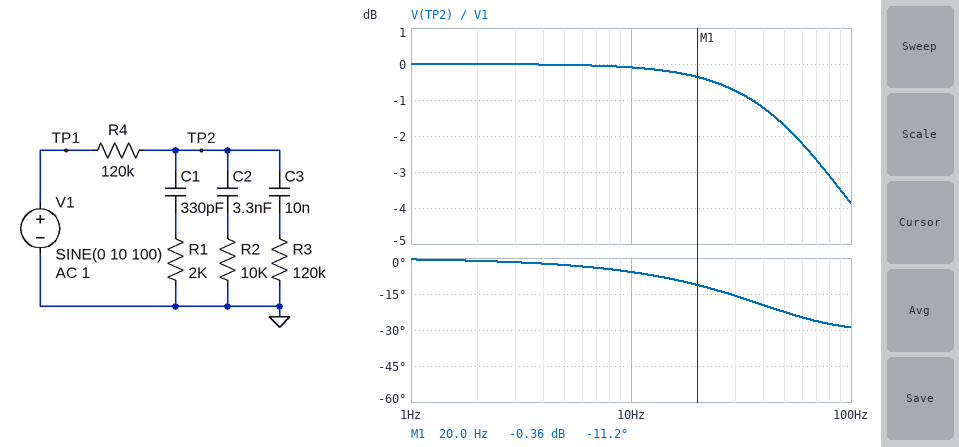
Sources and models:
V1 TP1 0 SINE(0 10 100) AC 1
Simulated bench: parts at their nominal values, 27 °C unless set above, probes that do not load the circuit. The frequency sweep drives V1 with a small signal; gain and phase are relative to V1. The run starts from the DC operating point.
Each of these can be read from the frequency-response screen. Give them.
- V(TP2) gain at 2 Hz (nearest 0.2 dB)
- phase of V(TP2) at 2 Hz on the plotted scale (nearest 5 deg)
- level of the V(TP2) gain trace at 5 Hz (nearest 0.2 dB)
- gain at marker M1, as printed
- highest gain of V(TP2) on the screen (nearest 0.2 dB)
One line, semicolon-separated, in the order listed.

0 dB; 0 deg; 0 dB; -0.36 dB; 0 dB
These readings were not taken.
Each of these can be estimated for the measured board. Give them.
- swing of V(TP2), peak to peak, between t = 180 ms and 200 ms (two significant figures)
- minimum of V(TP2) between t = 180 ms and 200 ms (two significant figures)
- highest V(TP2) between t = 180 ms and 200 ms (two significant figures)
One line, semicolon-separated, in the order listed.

13 V; -6.4 V; 6.4 V
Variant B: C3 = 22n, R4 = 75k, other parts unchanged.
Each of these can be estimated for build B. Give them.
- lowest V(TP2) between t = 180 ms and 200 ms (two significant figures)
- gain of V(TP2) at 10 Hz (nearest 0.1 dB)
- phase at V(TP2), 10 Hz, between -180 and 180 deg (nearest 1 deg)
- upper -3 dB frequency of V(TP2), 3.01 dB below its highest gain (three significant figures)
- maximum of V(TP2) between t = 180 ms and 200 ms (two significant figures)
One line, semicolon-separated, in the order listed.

-6.5 V; -0.2 dB; -7 deg; 67.4 Hz; 6.5 V
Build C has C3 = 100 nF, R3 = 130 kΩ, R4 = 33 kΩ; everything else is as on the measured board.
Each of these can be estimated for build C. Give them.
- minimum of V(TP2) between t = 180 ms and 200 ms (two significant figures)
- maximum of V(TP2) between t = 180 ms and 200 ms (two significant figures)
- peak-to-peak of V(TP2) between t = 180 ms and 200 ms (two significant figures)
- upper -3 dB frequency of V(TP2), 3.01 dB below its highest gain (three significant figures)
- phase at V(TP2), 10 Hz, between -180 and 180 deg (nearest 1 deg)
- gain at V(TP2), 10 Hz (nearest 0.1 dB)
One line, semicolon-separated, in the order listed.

-8.0 V; 8.0 V; 16 V; 684 Hz; -7 deg; -0.9 dB
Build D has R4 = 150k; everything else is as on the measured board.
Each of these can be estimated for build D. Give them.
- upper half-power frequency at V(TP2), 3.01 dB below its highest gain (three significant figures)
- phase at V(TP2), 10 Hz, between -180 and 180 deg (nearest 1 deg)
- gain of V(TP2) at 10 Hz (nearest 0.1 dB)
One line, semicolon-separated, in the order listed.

62.6 Hz; -7 deg; -0.1 dB
